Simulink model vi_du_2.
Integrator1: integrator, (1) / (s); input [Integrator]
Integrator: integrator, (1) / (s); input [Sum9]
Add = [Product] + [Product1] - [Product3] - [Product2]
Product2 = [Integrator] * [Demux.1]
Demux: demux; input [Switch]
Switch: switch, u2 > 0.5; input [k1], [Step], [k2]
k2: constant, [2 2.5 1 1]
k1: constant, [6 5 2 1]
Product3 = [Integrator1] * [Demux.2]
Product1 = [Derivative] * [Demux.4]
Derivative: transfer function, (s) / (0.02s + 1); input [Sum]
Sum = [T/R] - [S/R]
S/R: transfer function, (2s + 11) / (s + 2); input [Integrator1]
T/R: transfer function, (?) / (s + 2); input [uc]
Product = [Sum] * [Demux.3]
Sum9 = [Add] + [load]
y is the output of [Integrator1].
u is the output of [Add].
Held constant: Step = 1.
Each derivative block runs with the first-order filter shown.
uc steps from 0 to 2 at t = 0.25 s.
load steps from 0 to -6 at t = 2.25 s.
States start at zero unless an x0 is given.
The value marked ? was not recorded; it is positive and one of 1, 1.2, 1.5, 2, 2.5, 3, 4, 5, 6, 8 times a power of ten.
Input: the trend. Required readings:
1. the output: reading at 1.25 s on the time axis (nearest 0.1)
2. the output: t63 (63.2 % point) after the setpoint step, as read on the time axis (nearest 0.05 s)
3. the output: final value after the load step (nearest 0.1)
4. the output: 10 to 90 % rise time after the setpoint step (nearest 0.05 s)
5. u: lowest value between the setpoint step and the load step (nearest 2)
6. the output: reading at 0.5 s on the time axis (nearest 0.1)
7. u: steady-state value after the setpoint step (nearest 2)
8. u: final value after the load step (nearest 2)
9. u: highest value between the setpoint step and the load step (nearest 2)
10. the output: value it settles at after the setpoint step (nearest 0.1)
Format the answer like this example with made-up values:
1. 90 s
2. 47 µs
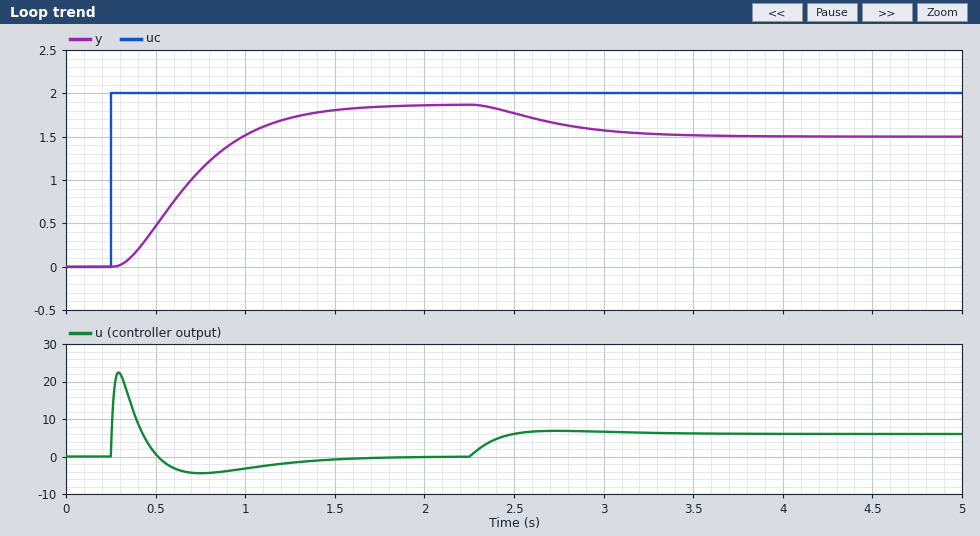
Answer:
1. 1.7
2. 0.80 s
3. 1.5
4. 0.80 s
5. -4
6. 0.5
7. 0
8. 6
9. 22
10. 1.9
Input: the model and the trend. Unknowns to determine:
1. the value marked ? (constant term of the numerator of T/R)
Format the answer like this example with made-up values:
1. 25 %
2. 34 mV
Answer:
1. 15
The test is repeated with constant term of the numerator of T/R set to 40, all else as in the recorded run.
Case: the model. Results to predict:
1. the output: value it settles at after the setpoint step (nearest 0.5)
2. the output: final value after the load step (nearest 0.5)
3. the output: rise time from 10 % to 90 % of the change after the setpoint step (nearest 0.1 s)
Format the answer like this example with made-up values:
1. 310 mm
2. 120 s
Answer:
1. 5.0
2. 4.5
3. 0.8 s
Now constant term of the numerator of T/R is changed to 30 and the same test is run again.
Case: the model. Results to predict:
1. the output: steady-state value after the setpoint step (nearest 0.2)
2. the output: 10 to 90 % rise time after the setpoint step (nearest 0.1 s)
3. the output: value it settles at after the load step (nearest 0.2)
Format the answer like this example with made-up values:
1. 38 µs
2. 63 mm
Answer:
1. 3.8
2. 0.8 s
3. 3.4
